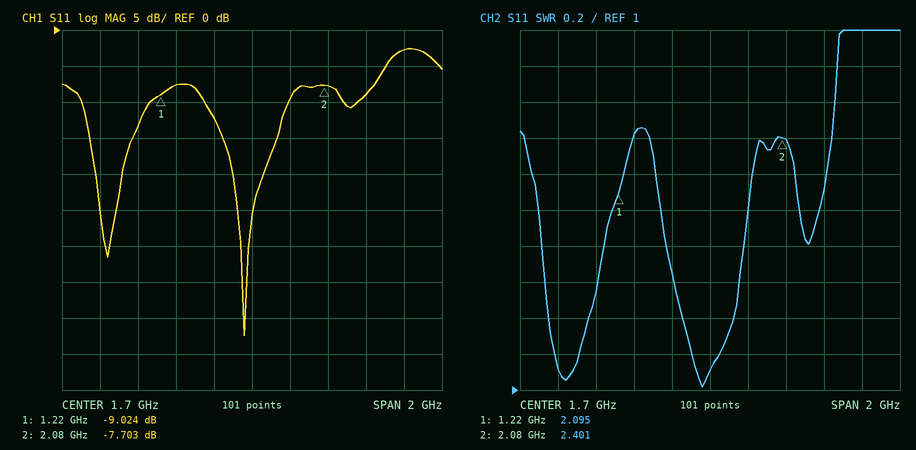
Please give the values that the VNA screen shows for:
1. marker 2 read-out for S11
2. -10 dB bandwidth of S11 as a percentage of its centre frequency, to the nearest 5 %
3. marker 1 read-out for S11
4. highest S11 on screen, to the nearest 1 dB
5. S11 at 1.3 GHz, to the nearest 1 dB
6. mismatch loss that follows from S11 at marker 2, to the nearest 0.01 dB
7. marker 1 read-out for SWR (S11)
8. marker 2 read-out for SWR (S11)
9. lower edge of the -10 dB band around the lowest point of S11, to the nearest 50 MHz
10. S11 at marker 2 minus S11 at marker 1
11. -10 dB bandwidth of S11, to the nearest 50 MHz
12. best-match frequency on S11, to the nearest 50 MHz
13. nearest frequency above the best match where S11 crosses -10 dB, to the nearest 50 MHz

-7.703 dB
25 %
-9.024 dB
-3 dB
-8 dB
0.81 dB
2.095
2.401
1.45 GHz
1.321 dB
450 MHz
1.65 GHz
1.90 GHz
